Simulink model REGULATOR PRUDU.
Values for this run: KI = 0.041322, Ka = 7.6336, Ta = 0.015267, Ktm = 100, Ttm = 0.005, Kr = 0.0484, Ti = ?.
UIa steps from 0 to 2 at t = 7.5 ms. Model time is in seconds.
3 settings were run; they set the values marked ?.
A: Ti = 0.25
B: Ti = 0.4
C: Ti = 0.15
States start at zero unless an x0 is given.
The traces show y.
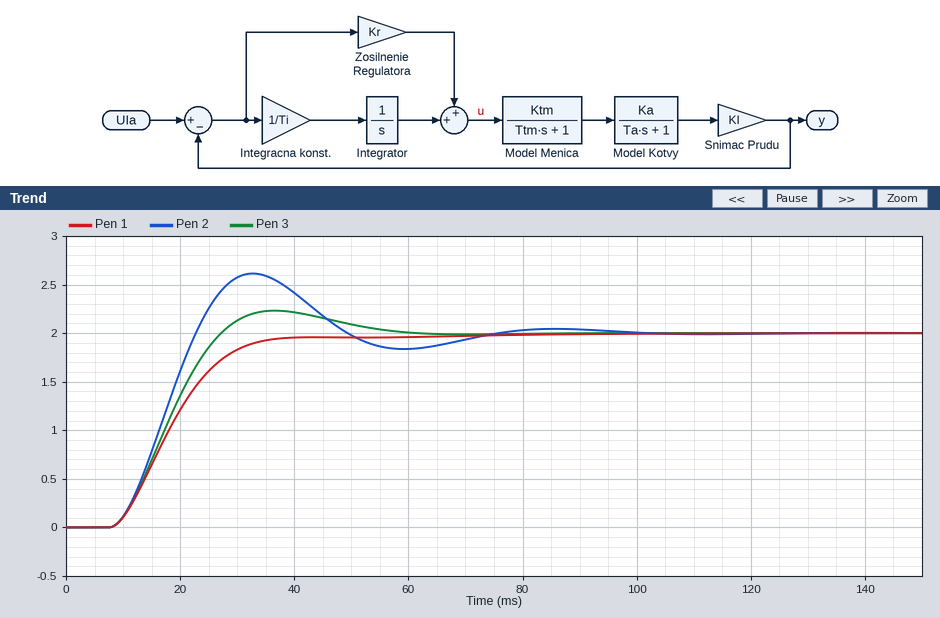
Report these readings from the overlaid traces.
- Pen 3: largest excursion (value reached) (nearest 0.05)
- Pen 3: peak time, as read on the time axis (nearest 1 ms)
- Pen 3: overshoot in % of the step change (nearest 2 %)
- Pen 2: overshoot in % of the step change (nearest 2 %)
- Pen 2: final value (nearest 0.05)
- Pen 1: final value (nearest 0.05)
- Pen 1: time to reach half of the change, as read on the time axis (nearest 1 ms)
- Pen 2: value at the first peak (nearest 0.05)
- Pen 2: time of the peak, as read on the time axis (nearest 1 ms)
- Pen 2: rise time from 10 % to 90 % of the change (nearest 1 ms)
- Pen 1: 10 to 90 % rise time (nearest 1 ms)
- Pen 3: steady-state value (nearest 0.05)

2.25
37 ms
12 %
30 %
2.00
2.00
18 ms
2.60
33 ms
10 ms
18 ms
2.00
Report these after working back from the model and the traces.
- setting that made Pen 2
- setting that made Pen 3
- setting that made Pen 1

C
A
B
